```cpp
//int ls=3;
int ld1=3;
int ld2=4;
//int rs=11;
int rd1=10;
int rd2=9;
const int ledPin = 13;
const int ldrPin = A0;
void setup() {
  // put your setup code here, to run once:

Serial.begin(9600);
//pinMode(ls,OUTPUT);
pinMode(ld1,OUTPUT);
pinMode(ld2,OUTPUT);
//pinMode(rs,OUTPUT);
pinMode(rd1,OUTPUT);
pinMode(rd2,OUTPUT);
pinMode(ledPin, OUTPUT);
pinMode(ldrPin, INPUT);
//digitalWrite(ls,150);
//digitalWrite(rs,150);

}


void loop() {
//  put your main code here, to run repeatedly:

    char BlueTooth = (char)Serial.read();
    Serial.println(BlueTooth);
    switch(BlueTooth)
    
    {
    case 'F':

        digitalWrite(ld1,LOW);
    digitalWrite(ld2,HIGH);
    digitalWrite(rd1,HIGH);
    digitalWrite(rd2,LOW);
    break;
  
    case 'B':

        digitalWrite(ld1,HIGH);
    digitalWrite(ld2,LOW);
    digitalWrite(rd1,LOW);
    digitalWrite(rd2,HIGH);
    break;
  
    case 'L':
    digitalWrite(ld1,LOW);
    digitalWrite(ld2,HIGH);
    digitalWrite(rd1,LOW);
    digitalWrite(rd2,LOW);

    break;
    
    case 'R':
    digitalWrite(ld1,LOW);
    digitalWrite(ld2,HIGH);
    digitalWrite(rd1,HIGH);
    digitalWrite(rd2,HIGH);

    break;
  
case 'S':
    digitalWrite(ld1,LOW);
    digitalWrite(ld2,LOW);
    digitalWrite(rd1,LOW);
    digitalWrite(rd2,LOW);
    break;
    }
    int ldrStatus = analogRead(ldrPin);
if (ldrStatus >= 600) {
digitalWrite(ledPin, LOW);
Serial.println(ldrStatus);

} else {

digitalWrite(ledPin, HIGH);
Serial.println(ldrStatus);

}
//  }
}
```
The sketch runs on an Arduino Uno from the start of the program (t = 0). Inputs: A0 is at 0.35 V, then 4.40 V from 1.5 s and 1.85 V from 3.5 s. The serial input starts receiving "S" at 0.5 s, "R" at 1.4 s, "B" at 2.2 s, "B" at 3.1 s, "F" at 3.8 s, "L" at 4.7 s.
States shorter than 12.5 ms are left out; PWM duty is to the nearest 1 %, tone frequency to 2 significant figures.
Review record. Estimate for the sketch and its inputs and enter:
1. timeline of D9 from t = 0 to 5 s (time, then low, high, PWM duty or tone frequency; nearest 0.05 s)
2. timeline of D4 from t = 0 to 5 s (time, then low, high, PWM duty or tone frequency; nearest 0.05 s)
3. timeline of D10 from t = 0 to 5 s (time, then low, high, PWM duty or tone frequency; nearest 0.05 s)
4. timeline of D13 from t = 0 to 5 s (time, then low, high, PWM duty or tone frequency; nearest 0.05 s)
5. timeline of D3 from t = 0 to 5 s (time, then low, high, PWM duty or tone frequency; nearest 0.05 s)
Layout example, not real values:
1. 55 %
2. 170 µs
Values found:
1. 0 s low; 1.4 s high; 3.8 s low
2. 0 s low; 1.4 s high; 2.2 s low; 3.8 s high
3. 0 s low; 1.4 s high; 2.2 s low; 3.8 s high; 4.7 s low
4. 0 s high; 1.5 s low; 3.5 s high
5. 0 s low; 2.2 s high; 3.8 s low
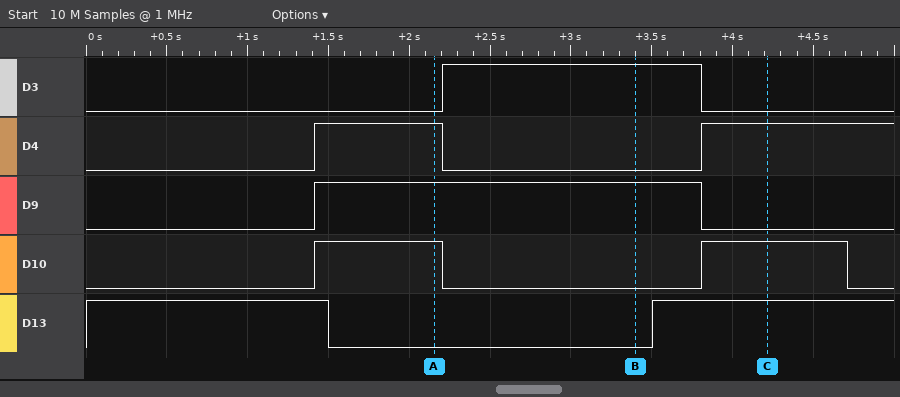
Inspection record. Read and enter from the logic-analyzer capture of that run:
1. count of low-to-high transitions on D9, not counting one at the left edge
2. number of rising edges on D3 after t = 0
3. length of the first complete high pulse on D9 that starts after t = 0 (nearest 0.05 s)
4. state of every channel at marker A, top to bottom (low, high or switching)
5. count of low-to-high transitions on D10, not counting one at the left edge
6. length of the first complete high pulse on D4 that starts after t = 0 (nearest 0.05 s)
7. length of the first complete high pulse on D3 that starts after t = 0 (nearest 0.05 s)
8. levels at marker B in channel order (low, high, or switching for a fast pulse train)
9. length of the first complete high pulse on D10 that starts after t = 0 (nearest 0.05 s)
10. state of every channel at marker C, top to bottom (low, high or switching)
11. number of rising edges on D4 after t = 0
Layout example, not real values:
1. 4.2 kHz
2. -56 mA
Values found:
1. 1
2. 1
3. 2.40 s
4. D3 low, D4 high, D9 high, D10 high, D13 low
5. 2
6. 0.80 s
7. 1.60 s
8. D3 high, D4 low, D9 high, D10 low, D13 low
9. 0.80 s
10. D3 low, D4 high, D9 low, D10 high, D13 high
11. 2
